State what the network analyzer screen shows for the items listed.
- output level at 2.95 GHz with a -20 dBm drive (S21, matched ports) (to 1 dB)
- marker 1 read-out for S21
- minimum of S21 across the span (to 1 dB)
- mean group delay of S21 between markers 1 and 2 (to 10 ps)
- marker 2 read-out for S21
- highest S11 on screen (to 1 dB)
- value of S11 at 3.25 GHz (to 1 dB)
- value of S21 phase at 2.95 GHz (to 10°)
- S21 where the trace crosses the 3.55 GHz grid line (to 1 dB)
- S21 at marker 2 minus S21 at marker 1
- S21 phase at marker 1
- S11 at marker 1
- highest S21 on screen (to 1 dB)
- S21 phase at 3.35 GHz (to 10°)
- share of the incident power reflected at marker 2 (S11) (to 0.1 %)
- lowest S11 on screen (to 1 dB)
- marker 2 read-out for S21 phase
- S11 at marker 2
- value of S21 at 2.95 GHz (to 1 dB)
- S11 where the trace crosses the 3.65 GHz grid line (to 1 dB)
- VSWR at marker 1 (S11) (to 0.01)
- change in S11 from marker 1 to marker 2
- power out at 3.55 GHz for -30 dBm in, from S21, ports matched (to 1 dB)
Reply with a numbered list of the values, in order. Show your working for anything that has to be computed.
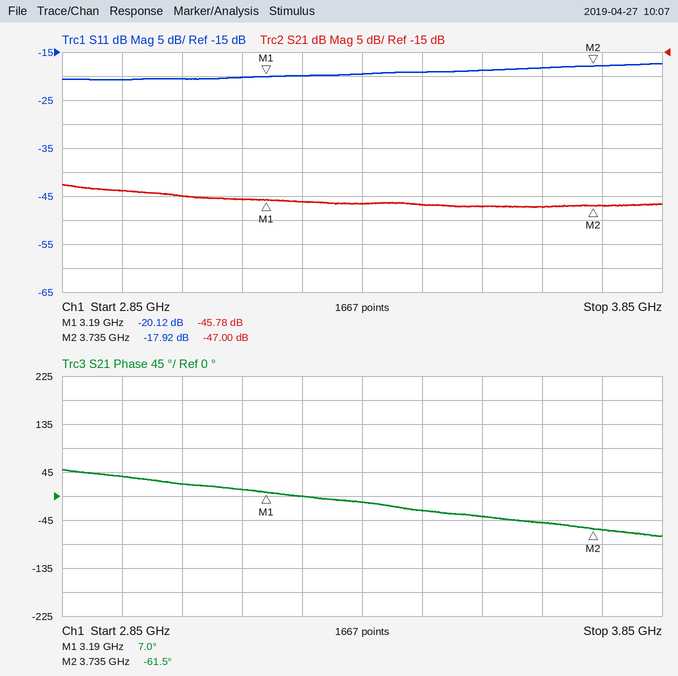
1. -20 dBm + (-44 dB) = -64 dBm
2. -45.78 dB
3. -47 dB
4. −(-61.5° − (7°))/(360° × 545 MHz) ≈ 349 ps, so 350 ps to the nearest 10 ps
5. -47.00 dB
6. -17 dB
7. -20 dB
8. 40°
9. -47 dB
10. -47 − (-45.78) = -1.22 dB
11. 7.0°
12. -20.12 dB
13. -43 dB
14. -10°
15. 10^(-17.92/10) ≈ 1.6 %
16. -21 dB
17. -61.5°
18. -17.92 dB
19. -44 dB
20. -18 dB
21. (1 + 0.0986)/(1 − 0.0986) ≈ 1.22
22. -17.92 − (-20.12) = 2.20 dB
23. -30 dBm + (-47 dB) = -77 dBm
